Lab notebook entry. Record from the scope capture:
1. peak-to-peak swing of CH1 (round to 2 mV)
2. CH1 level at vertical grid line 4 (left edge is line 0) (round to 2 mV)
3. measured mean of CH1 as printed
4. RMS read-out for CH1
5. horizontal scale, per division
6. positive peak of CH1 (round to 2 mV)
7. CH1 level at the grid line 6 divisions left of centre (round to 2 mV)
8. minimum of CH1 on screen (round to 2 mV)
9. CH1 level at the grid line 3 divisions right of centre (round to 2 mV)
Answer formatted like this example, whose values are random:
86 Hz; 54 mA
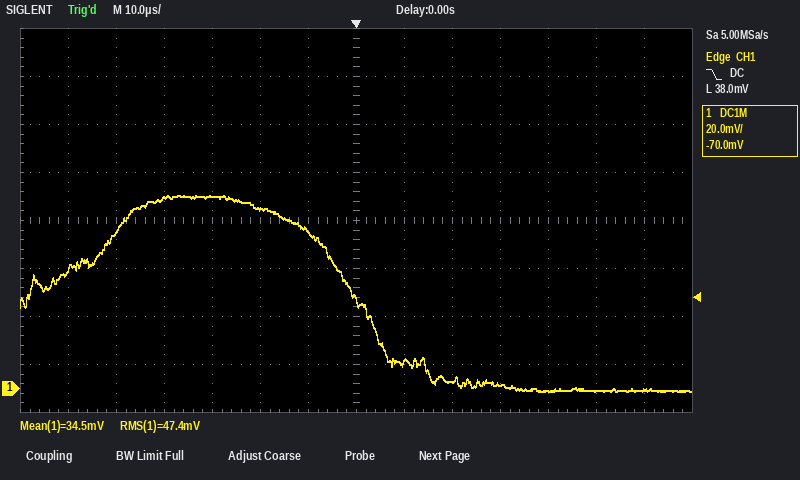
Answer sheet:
82 mV; 80 mV; 34.5 mV; 47.4 mV; 10 µs; 80 mV; 50 mV; -2 mV; 2 mV
